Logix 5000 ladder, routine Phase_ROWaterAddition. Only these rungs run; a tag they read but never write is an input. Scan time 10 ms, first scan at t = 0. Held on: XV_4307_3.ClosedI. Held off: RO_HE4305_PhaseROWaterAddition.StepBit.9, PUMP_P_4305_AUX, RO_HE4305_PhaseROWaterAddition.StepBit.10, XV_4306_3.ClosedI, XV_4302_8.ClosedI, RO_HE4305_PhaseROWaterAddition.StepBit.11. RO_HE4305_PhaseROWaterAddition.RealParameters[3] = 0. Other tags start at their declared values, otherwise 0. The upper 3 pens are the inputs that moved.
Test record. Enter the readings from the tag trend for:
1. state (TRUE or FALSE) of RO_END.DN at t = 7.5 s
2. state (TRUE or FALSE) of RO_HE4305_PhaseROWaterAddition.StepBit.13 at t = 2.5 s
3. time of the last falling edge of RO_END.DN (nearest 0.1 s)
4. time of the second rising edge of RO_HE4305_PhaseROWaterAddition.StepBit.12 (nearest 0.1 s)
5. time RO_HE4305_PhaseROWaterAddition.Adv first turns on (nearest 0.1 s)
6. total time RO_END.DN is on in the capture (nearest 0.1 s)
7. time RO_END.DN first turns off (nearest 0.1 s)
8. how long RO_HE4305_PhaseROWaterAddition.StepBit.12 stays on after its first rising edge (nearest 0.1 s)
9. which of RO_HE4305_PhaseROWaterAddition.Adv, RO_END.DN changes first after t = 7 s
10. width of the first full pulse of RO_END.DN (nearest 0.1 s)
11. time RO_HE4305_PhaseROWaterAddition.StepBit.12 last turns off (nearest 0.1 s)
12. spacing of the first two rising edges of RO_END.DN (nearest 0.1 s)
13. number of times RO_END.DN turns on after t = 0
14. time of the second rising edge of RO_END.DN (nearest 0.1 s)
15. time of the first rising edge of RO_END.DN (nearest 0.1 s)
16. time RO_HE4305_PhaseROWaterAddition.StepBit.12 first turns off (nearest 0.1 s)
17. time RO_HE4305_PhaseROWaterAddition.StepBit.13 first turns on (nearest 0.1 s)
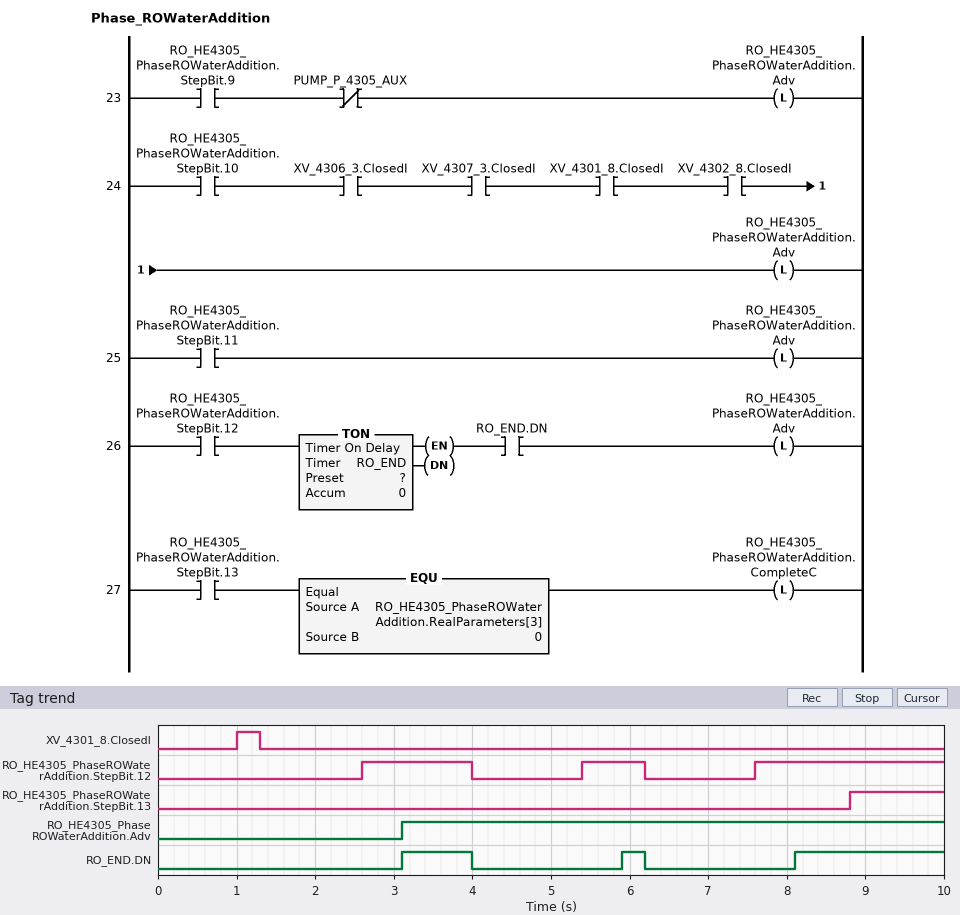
FALSE
FALSE
6.2 s
5.4 s
3.1 s
3.1 s
4.0 s
1.4 s
RO_END.DN
0.9 s
6.2 s
2.8 s
3
5.9 s
3.1 s
4.0 s
8.8 s
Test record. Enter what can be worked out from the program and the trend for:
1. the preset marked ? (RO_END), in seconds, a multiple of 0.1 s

0.5 s
